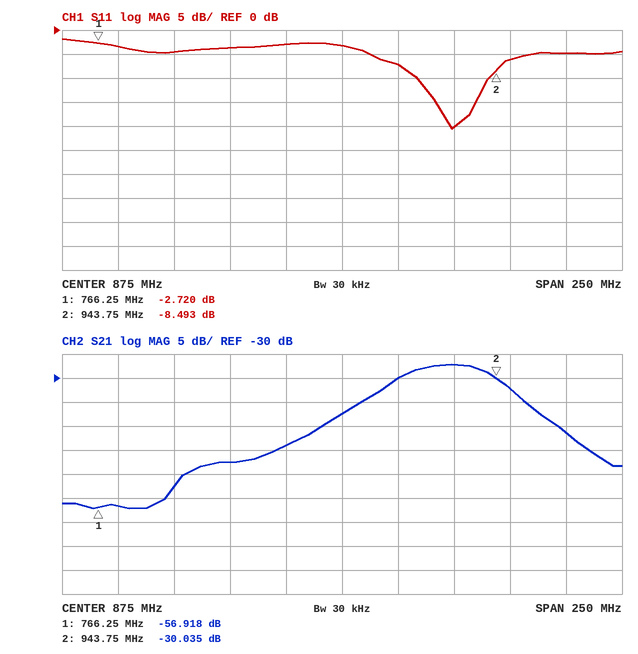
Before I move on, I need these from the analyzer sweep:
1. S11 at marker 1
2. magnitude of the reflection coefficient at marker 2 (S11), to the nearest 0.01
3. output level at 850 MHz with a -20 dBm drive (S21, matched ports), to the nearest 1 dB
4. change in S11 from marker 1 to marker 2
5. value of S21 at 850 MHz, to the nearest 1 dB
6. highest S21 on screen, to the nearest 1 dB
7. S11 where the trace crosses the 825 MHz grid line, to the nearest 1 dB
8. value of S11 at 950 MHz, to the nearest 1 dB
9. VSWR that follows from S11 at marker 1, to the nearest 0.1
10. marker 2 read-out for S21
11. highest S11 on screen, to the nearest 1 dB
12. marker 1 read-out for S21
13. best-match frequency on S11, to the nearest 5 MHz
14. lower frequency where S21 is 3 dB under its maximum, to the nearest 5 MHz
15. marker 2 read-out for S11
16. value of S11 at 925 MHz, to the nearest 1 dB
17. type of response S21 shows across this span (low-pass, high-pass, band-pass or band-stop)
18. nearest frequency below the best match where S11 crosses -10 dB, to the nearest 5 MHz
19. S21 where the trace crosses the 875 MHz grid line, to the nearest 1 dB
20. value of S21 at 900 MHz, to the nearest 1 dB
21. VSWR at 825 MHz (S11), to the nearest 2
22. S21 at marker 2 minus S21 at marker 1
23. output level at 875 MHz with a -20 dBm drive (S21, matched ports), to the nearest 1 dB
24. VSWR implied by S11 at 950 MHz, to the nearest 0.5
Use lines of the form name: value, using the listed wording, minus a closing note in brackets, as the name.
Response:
S11 at marker 1: -2.720 dB
magnitude of the reflection coefficient at marker 2 (S11), to the nearest 0.01: 0.38
output level at 850 MHz with a -20 dBm drive (S21, matched ports), to the nearest 1 dB: -64 dBm
change in S11 from marker 1 to marker 2: -5.773 dB
value of S21 at 850 MHz, to the nearest 1 dB: -44 dB
highest S21 on screen, to the nearest 1 dB: -27 dB
S11 where the trace crosses the 825 MHz grid line, to the nearest 1 dB: -4 dB
value of S11 at 950 MHz, to the nearest 1 dB: -6 dB
VSWR that follows from S11 at marker 1, to the nearest 0.1: 6.4
marker 2 read-out for S21: -30.035 dB
highest S11 on screen, to the nearest 1 dB: -2 dB
marker 1 read-out for S21: -56.918 dB
best-match frequency on S11, to the nearest 5 MHz: 925 MHz
lower frequency where S21 is 3 dB under its maximum, to the nearest 5 MHz: 900 MHz
marker 2 read-out for S11: -8.493 dB
value of S11 at 925 MHz, to the nearest 1 dB: -20 dB
type of response S21 shows across this span: band-pass
nearest frequency below the best match where S11 crosses -10 dB, to the nearest 5 MHz: 910 MHz
S21 where the trace crosses the 875 MHz grid line, to the nearest 1 dB: -37 dB
value of S21 at 900 MHz, to the nearest 1 dB: -30 dB
VSWR at 825 MHz (S11), to the nearest 2: 4
S21 at marker 2 minus S21 at marker 1: 26.883 dB
output level at 875 MHz with a -20 dBm drive (S21, matched ports), to the nearest 1 dB: -57 dBm
VSWR implied by S11 at 950 MHz, to the nearest 0.5: 3.0
